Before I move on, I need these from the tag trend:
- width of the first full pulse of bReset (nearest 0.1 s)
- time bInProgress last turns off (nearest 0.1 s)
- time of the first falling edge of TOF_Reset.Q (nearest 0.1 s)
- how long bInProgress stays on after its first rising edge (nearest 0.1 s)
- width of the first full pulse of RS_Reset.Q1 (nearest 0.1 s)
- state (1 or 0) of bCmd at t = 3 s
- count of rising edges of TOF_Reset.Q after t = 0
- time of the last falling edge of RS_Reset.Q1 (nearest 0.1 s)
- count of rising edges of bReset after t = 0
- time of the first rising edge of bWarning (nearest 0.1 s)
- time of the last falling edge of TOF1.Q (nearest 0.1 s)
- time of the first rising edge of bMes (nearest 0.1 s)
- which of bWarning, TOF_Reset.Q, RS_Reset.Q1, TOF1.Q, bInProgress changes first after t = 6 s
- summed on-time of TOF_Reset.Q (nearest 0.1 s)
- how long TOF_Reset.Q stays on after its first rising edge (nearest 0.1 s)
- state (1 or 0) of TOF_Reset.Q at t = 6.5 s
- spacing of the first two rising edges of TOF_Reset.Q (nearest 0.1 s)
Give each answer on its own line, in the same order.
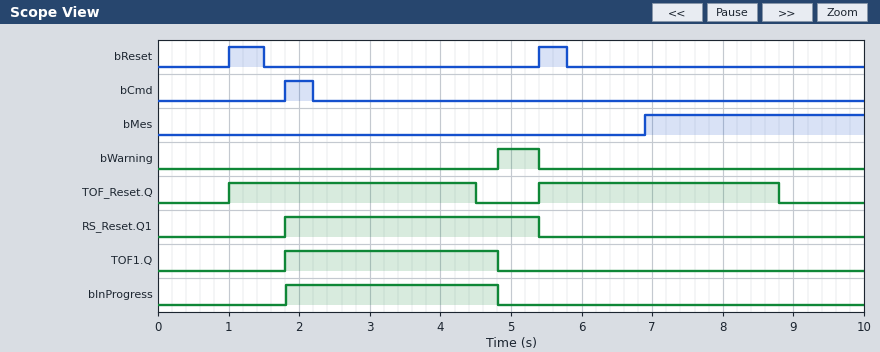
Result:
0.5 s
4.8 s
4.5 s
3.0 s
3.6 s
0
2
5.4 s
2
4.8 s
4.8 s
6.9 s
TOF_Reset.Q
6.9 s
3.5 s
1
4.4 s
